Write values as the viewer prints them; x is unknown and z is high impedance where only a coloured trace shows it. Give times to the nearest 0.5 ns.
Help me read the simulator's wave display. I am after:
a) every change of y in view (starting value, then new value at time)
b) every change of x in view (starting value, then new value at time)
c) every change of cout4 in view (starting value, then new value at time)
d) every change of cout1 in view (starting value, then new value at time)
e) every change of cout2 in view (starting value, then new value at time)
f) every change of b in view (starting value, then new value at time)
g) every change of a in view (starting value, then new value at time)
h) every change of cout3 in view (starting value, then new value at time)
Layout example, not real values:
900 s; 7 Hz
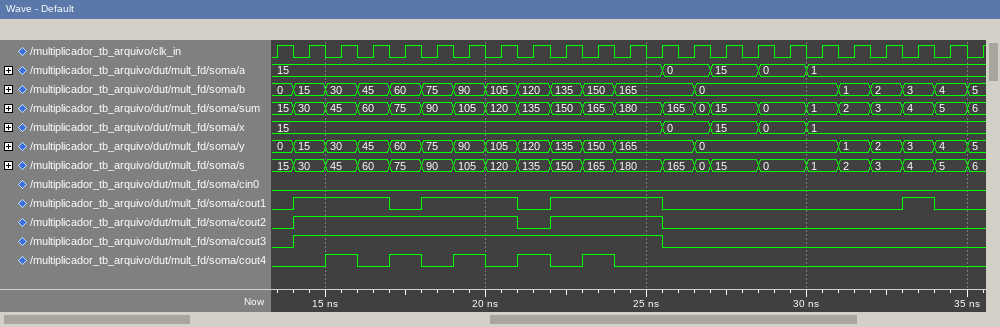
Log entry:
0, 15 at 14 ns, 30 at 15 ns, 45 at 16 ns, 60 at 17 ns, 75 at 18 ns, 90 at 19 ns, 105 at 20 ns, 120 at 21 ns, 135 at 22 ns, 150 at 23 ns, 165 at 24 ns, 0 at 26.5 ns, 1 at 31 ns, 2 at 32 ns, 3 at 33 ns, 4 at 34 ns, 5 at 35 ns; 15, 0 at 25.5 ns, 15 at 27 ns, 0 at 28.5 ns, 1 at 30 ns; 0, 1 at 15 ns, 0 at 16 ns, 1 at 17 ns, 0 at 18 ns, 1 at 19 ns, 0 at 20 ns, 1 at 21 ns, 0 at 22 ns, 1 at 23 ns, 0 at 24 ns; 0, 1 at 14 ns, 0 at 17 ns, 1 at 18 ns, 0 at 21 ns, 1 at 22 ns, 0 at 25.5 ns, 1 at 33 ns, 0 at 34 ns; 0, 1 at 14 ns, 0 at 21 ns, 1 at 22 ns, 0 at 25.5 ns; 0, 15 at 14 ns, 30 at 15 ns, 45 at 16 ns, 60 at 17 ns, 75 at 18 ns, 90 at 19 ns, 105 at 20 ns, 120 at 21 ns, 135 at 22 ns, 150 at 23 ns, 165 at 24 ns, 0 at 26.5 ns, 1 at 31 ns, 2 at 32 ns, 3 at 33 ns, 4 at 34 ns, 5 at 35 ns; 15, 0 at 25.5 ns, 15 at 27 ns, 0 at 28.5 ns, 1 at 30 ns; 0, 1 at 14 ns, 0 at 25.5 ns
